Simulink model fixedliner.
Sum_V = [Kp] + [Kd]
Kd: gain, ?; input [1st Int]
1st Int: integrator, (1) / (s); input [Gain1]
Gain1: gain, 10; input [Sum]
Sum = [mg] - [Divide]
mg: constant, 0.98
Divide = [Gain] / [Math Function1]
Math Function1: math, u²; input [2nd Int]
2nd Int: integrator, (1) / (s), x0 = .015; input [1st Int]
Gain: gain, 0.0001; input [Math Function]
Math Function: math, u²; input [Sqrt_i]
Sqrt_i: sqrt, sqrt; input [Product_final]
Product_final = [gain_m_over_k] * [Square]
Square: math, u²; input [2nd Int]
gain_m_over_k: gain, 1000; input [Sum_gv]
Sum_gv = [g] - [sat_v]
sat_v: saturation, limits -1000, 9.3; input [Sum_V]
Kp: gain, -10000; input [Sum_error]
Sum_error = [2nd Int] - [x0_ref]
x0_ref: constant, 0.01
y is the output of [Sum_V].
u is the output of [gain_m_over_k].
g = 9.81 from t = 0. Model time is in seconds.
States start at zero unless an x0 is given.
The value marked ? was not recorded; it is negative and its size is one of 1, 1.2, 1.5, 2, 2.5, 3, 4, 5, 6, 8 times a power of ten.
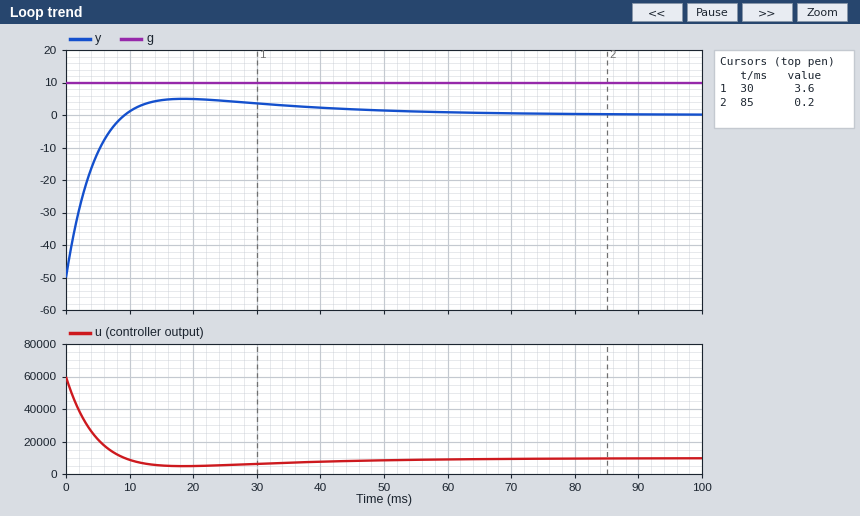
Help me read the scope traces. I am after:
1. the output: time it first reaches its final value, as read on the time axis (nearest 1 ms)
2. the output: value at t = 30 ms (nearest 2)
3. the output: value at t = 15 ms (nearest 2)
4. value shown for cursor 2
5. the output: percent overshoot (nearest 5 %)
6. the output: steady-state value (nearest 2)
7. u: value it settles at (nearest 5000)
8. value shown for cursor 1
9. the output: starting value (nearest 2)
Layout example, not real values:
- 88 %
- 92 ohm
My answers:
- 9 ms
- 4
- 4
- 0.2
- 10 %
- 0
- 10000
- 3.6
- -50
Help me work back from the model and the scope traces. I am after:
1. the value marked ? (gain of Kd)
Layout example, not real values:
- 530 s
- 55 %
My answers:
- -250
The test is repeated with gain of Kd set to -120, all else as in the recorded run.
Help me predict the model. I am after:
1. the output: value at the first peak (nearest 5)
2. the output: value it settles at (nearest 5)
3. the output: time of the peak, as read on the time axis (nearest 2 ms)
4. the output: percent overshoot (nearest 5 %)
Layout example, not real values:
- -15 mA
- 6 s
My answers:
- 15
- 0
- 28 ms
- 30 %
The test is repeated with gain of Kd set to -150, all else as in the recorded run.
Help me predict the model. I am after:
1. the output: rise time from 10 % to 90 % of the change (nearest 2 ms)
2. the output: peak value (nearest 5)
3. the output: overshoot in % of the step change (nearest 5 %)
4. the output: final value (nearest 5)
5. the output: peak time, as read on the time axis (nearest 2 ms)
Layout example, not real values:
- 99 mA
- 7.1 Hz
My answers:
- 8 ms
- 10
- 20 %
- 0
- 22 ms
